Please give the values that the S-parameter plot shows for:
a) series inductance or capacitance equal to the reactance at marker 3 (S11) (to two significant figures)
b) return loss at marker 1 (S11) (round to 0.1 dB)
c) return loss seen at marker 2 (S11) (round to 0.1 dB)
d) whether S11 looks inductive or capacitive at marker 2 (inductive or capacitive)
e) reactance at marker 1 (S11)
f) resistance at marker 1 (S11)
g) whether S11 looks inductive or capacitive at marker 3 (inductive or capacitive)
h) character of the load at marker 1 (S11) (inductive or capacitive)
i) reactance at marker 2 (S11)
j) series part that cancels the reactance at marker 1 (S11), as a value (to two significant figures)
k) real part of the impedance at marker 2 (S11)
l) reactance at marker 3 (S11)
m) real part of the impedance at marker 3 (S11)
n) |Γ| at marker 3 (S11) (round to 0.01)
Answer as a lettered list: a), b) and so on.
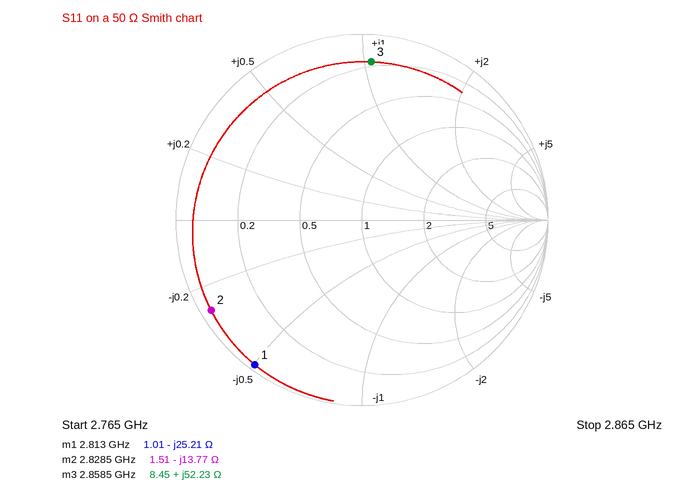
a) 2.9 nH
b) 0.3 dB
c) 0.5 dB
d) capacitive
e) -25.21 Ω
f) 1.01 Ω
g) inductive
h) capacitive
i) -13.77 Ω
j) 1.4 nH
k) 1.51 Ω
l) +52.23 Ω
m) 8.45 Ω
n) 0.85
